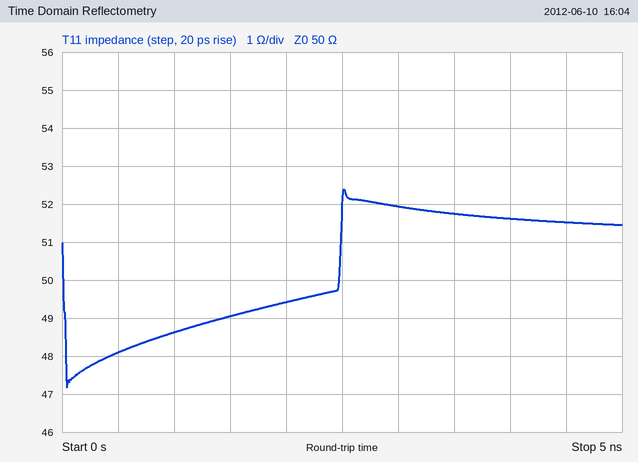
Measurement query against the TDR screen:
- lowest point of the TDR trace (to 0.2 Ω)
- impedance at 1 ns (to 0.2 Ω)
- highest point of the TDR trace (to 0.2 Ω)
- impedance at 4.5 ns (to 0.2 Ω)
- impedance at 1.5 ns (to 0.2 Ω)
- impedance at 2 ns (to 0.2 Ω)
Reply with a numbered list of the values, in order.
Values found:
1. 47.2 Ω
2. 48.6 Ω
3. 52.4 Ω
4. 51.6 Ω
5. 49.0 Ω
6. 49.4 Ω
